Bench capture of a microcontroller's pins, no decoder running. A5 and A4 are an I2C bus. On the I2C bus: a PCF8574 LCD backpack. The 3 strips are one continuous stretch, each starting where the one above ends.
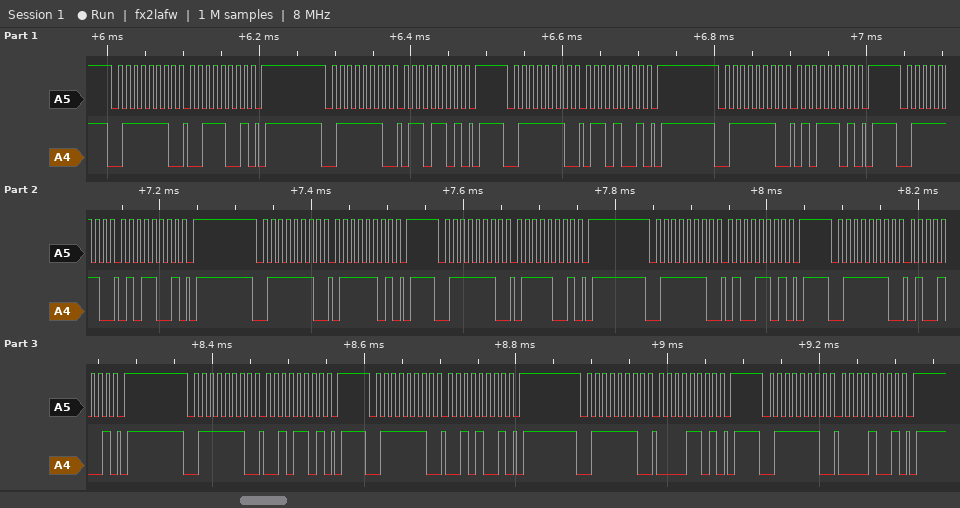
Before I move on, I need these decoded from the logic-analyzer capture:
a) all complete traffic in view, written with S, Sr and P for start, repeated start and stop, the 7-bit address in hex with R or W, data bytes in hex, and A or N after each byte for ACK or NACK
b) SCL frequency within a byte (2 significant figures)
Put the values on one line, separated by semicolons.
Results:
S 3FW A 39 A P S 3FW A 6D A P S 3FW A 69 A P S 3FW A 5D A P S 3FW A 59 A P S 3FW A 7D A P S 3FW A 79 A P S 3FW A 4D A P S 3FW A 49 A P S 3FW A 2D A P S 3FW A 29 A P S 3FW A 0D A P S 3FW A 09 A P; 100 kHz
